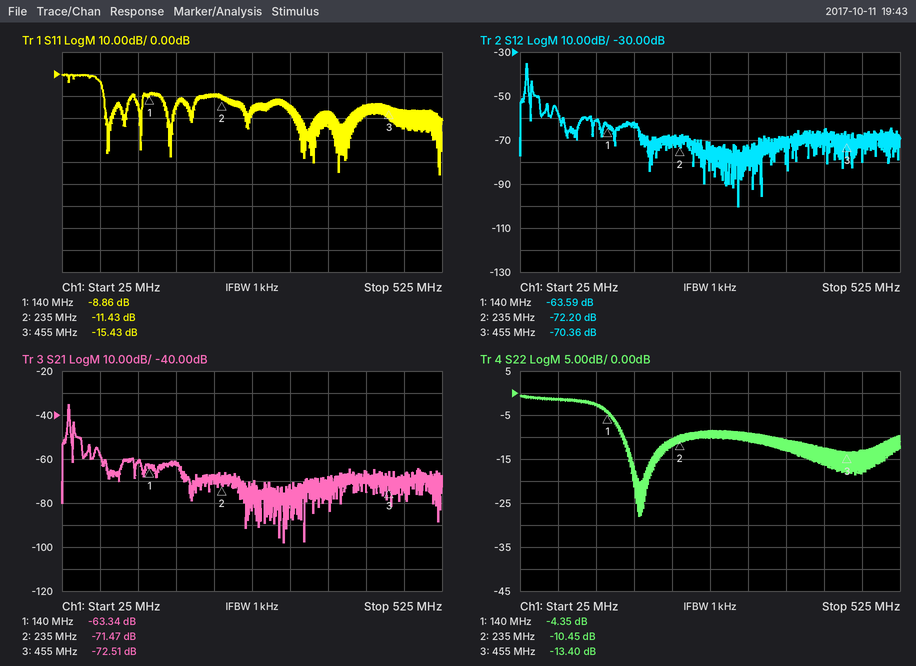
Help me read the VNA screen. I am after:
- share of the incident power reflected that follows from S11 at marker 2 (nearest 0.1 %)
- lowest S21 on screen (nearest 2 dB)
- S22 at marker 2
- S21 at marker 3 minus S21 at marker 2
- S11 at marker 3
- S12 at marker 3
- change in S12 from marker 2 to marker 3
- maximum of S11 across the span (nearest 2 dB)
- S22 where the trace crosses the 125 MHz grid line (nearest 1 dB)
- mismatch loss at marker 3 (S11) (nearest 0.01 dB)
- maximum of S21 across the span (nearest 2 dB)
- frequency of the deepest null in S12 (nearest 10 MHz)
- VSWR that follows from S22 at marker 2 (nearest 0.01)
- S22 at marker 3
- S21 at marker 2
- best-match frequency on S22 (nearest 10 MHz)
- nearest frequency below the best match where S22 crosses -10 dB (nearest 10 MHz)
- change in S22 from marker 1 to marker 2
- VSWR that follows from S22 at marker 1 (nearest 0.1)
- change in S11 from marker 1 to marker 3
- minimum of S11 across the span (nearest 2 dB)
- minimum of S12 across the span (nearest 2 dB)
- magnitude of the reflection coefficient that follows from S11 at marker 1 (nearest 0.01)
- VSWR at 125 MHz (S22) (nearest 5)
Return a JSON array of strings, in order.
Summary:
["7.2 %", "-98 dB", "-10.45 dB", "-1.04 dB", "-15.43 dB", "-70.36 dB", "1.84 dB", "0 dB", "-3 dB", "0.13 dB", "-36 dB", "310 MHz", "1.86", "-13.40 dB", "-71.47 dB", "180 MHz", "160 MHz", "-6.10 dB", "4.1", "-6.57 dB", "-46 dB", "-100 dB", "0.36", "5"]
